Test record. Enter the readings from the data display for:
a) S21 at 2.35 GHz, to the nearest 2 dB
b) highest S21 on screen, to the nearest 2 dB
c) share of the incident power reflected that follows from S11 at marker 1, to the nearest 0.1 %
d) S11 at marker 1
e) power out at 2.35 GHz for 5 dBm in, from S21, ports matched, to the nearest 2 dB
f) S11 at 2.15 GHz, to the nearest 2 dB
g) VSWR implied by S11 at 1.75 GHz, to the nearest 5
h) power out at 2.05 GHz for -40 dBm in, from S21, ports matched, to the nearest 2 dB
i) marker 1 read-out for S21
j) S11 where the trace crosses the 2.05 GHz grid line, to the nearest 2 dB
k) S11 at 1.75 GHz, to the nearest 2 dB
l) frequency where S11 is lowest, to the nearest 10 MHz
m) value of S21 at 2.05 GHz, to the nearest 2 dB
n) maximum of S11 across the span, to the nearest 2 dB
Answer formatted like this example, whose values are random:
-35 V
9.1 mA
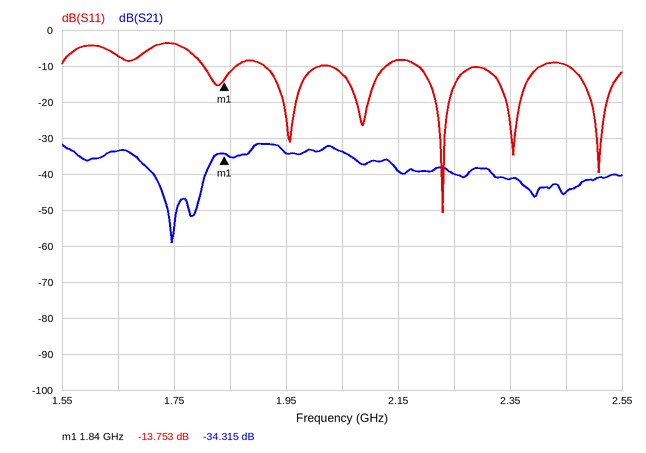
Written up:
-42 dB
-32 dB
4.2 %
-13.753 dB
-36 dBm
-8 dB
5
-74 dBm
-34.315 dB
-12 dB
-4 dB
2.23 GHz
-34 dB
-4 dB
